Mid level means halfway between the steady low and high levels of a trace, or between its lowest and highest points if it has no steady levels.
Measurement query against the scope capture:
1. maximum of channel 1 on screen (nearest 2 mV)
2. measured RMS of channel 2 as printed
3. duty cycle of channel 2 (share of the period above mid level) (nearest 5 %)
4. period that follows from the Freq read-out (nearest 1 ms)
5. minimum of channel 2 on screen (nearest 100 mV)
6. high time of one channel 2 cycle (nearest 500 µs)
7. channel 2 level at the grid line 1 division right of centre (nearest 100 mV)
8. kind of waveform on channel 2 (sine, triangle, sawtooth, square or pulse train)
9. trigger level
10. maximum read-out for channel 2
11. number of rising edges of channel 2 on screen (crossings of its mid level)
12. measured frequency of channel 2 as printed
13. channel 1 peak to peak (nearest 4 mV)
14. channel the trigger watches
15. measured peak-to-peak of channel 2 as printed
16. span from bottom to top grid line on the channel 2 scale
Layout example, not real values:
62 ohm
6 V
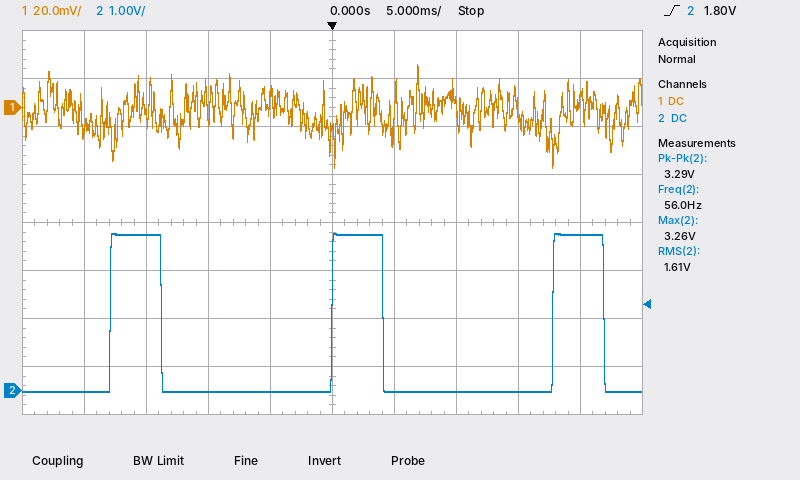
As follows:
18 mV
1.61 V
25 %
18 ms
0.0 V
4.0 ms
0.0 V
pulse train
1.80 V
3.26 V
3
56.0 Hz
44 mV
channel 2
3.29 V
8 V
